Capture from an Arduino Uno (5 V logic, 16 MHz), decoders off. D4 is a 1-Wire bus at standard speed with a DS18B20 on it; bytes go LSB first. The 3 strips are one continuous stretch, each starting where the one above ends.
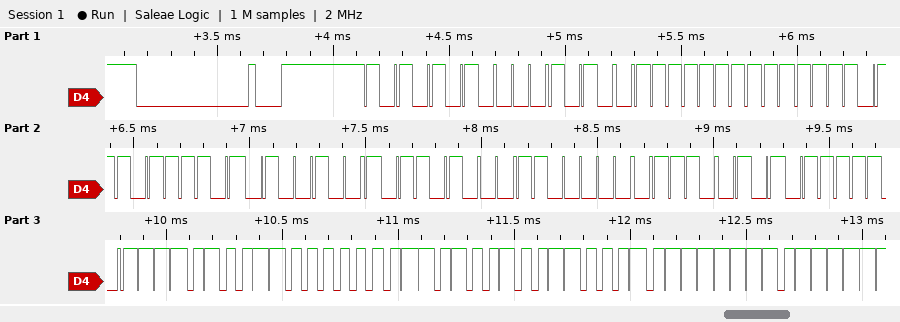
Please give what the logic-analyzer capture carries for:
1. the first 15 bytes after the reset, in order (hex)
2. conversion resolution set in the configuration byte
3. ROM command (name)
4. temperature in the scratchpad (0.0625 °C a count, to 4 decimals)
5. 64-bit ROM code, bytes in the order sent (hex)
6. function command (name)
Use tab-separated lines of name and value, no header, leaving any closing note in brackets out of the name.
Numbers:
the first 15 bytes after the reset, in order	55 28 FF BF BD 92 16 03 A7 BE 97 01 4B 46 7F
conversion resolution set in the configuration byte	12 bits
ROM command	Match ROM
temperature in the scratchpad	25.4375 °C
64-bit ROM code, bytes in the order sent	28 FF BF BD 92 16 03 A7
function command	Read Scratchpad
